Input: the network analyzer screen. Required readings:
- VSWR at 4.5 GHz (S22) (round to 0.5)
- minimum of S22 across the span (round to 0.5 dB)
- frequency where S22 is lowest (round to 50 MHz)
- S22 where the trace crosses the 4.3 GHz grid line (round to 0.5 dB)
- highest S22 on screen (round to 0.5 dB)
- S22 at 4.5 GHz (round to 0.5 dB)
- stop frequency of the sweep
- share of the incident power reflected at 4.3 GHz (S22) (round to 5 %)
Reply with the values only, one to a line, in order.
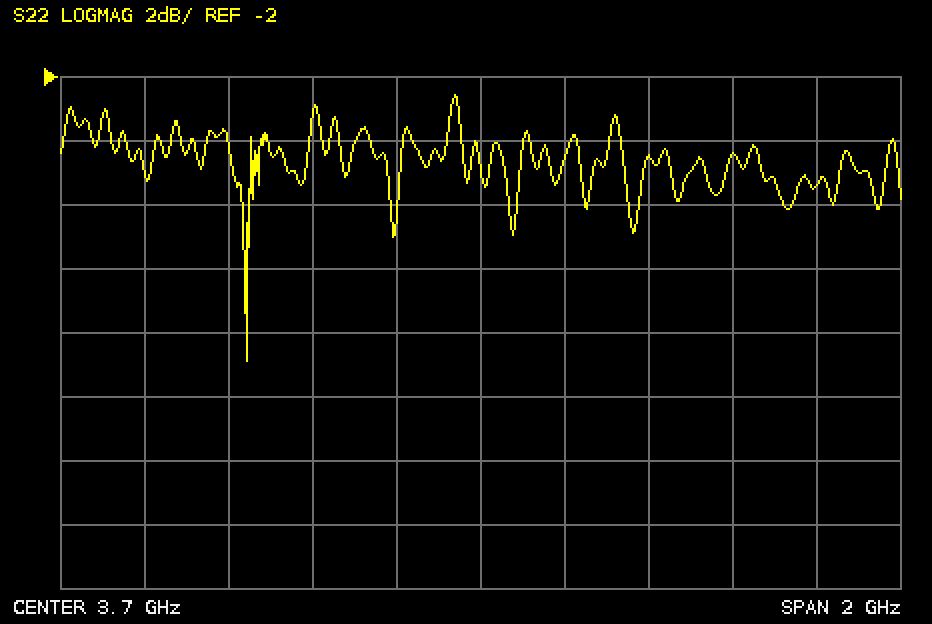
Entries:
3.5
-11.0 dB
3.15 GHz
-4.5 dB
-2.5 dB
-5.5 dB
4.7 GHz
35 %
